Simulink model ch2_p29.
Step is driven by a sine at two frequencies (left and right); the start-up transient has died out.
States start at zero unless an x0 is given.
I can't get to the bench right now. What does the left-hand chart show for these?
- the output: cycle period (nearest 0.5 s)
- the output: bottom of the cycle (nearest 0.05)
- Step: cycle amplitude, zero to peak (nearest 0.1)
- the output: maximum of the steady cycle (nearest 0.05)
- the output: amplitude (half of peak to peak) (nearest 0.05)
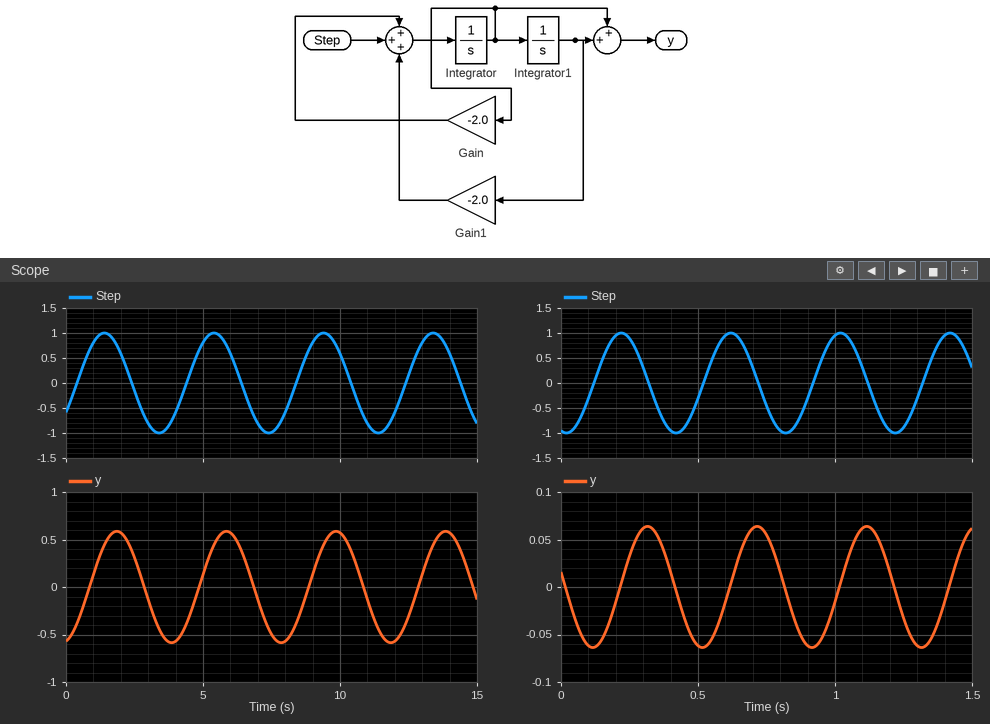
4.0 s
-0.60
1.0
0.60
0.60
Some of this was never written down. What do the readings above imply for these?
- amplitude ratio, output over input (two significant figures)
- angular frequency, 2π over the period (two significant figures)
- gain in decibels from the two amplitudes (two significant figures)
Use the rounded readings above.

0.60
1.6 rad/s
-4.4 dB
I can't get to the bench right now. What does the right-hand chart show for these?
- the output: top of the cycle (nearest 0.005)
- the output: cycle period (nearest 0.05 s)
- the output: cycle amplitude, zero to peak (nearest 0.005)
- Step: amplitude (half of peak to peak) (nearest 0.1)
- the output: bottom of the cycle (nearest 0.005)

0.065
0.40 s
0.065
1.0
-0.065
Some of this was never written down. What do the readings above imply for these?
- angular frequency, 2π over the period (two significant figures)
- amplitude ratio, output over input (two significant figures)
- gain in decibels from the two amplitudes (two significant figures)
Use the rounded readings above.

16 rad/s
0.065
-24 dB
